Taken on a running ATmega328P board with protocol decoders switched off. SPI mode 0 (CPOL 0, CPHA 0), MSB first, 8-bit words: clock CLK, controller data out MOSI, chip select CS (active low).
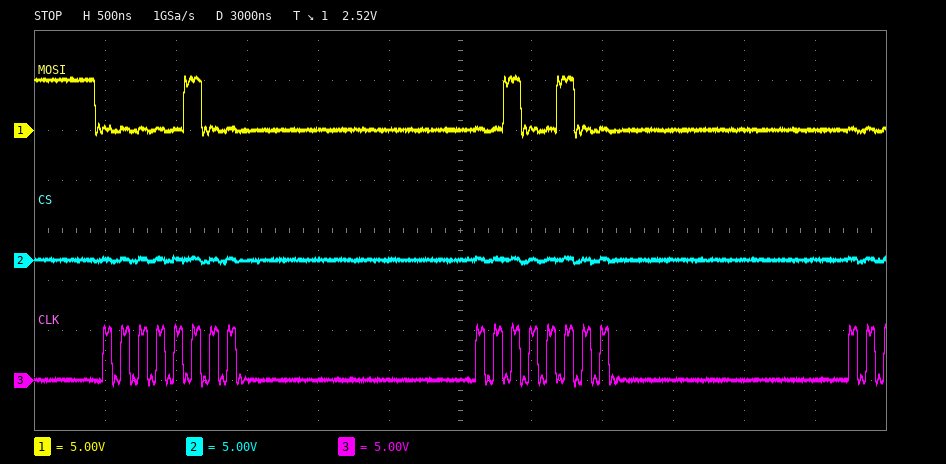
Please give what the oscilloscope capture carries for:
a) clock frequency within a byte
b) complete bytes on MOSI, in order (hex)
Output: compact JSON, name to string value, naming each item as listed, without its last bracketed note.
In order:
{"clock frequency within a byte": "8 MHz", "complete bytes on MOSI, in order": "04 24"}
